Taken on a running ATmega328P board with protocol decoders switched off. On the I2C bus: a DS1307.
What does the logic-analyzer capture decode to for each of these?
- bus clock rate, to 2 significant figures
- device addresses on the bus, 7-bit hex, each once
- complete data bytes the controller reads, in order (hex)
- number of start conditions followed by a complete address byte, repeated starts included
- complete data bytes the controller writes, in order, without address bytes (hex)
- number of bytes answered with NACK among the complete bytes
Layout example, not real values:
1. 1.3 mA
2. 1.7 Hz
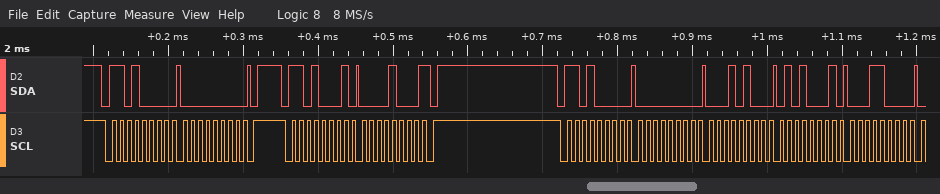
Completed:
1. 100 kHz
2. 0x68
3. 08
4. 3
5. 00 00 14 51 18
6. 1
